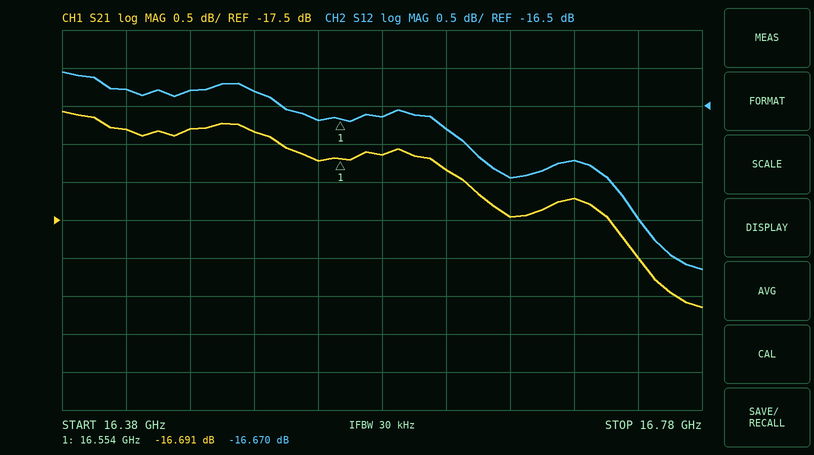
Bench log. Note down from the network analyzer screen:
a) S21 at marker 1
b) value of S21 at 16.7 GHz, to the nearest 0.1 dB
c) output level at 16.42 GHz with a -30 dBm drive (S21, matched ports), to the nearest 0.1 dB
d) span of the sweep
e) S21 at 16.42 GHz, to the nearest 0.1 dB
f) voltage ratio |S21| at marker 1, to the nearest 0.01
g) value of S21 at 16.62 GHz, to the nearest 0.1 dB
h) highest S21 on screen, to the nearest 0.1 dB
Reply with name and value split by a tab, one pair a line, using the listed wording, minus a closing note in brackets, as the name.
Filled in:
S21 at marker 1	-16.691 dB
value of S21 at 16.7 GHz, to the nearest 0.1 dB	-17.2 dB
output level at 16.42 GHz with a -30 dBm drive (S21, matched ports), to the nearest 0.1 dB	-46.3 dBm
span of the sweep	400 MHz
S21 at 16.42 GHz, to the nearest 0.1 dB	-16.3 dB
voltage ratio |S21| at marker 1, to the nearest 0.01	0.15
value of S21 at 16.62 GHz, to the nearest 0.1 dB	-16.8 dB
highest S21 on screen, to the nearest 0.1 dB	-16.1 dB
